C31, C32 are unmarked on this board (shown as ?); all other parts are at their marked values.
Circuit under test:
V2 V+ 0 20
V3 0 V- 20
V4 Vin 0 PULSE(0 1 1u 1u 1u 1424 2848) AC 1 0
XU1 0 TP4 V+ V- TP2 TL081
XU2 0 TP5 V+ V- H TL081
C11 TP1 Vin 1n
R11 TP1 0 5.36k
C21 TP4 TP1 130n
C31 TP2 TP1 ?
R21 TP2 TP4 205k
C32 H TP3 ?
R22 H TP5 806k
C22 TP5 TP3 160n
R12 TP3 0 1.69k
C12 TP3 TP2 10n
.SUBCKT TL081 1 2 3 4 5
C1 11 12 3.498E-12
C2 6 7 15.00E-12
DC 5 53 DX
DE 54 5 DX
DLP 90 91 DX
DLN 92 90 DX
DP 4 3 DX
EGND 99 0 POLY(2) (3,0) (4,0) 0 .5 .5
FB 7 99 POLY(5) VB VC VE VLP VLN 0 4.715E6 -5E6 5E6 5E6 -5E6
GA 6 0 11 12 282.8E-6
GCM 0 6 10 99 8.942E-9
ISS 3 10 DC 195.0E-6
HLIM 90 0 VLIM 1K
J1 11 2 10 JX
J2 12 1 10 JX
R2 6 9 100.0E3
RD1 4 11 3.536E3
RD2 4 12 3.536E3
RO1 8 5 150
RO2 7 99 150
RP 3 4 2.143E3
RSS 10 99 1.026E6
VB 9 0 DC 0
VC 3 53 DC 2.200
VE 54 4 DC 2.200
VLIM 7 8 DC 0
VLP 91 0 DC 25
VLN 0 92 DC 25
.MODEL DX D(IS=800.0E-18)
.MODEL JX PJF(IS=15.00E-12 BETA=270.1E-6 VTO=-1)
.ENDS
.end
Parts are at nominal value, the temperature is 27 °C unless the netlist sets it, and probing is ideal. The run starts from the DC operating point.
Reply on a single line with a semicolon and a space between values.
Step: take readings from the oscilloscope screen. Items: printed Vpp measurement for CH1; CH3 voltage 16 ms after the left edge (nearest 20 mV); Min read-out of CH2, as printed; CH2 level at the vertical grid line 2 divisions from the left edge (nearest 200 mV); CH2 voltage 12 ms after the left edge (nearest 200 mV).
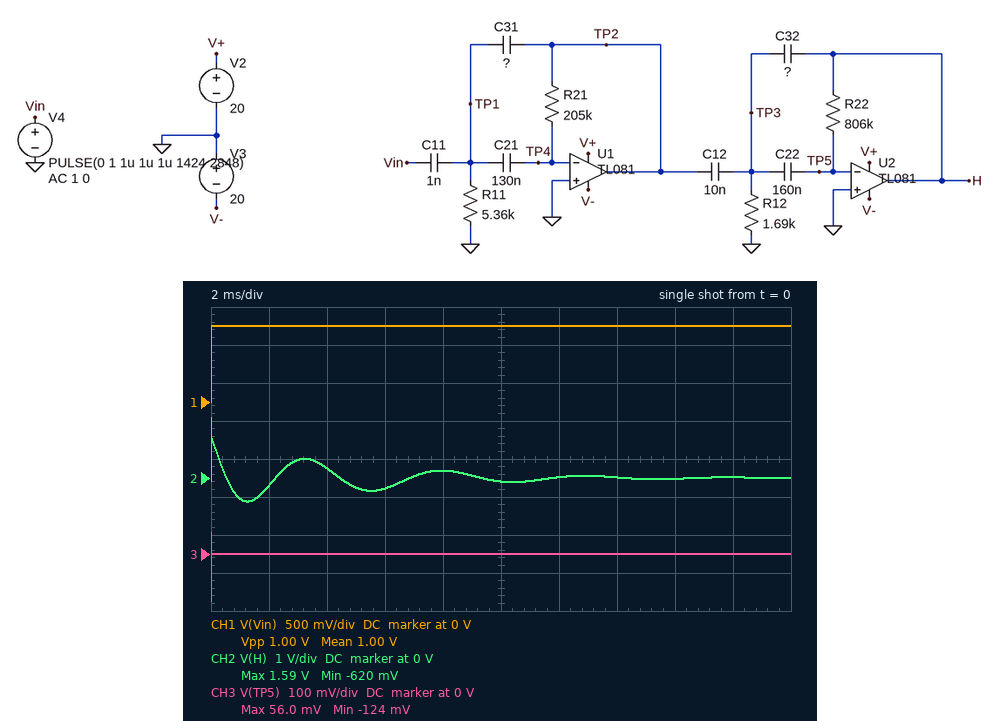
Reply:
1.00 V; 0 V; -620 mV; 200 mV; 0 V
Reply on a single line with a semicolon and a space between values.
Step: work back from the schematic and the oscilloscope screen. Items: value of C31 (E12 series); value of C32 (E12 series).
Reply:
3.3 nF; 2.7 nF
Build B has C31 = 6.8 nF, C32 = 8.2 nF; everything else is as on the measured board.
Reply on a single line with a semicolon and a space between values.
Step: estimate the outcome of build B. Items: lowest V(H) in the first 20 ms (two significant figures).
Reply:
-120 mV
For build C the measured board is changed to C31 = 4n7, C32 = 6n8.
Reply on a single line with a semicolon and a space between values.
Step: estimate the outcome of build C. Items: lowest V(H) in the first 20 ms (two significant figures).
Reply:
-180 mV
